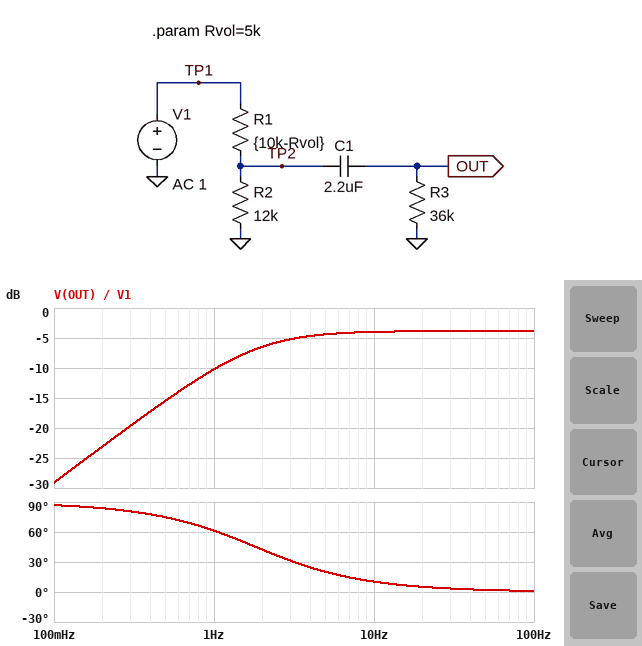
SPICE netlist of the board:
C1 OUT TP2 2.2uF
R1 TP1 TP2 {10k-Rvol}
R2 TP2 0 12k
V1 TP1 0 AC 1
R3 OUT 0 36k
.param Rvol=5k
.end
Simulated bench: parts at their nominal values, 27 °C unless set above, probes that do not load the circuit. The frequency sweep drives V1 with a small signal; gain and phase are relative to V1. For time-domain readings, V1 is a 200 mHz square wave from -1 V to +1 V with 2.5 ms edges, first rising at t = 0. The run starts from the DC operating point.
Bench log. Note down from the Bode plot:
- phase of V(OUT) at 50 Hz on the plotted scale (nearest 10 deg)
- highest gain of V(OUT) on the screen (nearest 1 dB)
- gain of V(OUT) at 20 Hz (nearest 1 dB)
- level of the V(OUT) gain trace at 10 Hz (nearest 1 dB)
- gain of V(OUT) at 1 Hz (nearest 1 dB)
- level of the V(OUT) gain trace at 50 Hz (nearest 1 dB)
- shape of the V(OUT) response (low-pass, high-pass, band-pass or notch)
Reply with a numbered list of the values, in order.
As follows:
1. 0 deg
2. -4 dB
3. -4 dB
4. -4 dB
5. -10 dB
6. -4 dB
7. high-pass
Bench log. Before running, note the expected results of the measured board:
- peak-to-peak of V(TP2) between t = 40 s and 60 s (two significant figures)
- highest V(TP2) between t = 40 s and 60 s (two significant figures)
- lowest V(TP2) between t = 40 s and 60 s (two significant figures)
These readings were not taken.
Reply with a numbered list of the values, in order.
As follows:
1. 1.4 V
2. 710 mV
3. -710 mV
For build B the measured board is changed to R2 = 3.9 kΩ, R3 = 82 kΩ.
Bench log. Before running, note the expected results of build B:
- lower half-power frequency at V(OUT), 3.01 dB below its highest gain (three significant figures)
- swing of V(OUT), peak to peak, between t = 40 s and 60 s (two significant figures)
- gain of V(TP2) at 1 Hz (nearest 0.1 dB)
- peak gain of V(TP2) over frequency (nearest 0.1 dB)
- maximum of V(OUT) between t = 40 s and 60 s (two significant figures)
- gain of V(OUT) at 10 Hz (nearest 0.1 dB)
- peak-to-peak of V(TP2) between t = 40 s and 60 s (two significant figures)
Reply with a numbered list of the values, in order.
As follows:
1. 859 mHz
2. 1.7 V
3. -7.3 dB
4. -7.2 dB
5. 850 mV
6. -7.4 dB
7. 880 mV
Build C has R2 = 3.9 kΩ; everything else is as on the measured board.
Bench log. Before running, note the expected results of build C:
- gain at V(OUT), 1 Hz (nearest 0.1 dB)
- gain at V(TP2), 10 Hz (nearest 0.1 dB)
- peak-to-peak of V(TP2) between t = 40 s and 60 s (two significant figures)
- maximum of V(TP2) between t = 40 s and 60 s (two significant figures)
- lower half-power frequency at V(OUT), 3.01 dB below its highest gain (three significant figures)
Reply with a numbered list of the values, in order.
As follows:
1. -14.3 dB
2. -7.7 dB
3. 880 mV
4. 440 mV
5. 1.89 Hz
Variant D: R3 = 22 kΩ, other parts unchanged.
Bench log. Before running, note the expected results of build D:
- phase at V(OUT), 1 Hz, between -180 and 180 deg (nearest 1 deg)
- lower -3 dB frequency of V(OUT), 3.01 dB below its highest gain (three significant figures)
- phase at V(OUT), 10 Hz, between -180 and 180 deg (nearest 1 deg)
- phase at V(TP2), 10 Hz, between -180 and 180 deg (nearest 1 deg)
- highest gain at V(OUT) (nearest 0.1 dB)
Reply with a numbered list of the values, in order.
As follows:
1. 71 deg
2. 2.83 Hz
3. 16 deg
4. -2 deg
5. -4.3 dB
